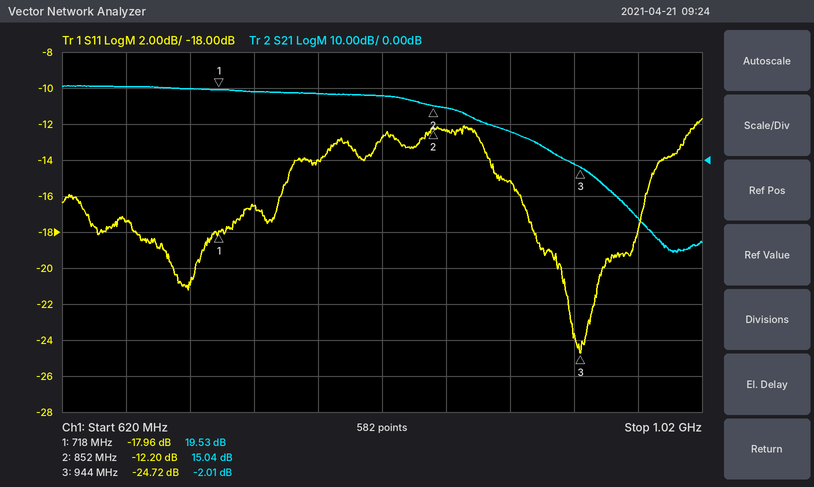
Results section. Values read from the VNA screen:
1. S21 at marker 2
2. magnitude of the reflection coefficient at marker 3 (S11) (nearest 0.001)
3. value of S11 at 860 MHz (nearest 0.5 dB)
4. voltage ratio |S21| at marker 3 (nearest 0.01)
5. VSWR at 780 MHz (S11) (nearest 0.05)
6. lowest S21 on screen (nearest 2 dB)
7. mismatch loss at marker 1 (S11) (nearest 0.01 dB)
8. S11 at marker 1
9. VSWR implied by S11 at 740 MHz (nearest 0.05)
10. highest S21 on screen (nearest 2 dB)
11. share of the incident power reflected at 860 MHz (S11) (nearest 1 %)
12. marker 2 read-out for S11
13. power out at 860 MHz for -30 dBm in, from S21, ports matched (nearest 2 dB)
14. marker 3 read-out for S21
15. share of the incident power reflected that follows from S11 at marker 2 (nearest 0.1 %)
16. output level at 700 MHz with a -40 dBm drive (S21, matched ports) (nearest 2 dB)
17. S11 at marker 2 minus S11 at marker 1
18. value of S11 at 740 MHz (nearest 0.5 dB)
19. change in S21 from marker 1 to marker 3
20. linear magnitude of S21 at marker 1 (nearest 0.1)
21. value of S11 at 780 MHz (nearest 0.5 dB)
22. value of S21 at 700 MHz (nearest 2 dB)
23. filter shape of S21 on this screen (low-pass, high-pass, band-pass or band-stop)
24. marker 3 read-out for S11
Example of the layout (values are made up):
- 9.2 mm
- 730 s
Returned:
- 15.04 dB
- 0.058
- -12.5 dB
- 0.79
- 1.50
- -26 dB
- 0.07 dB
- -17.96 dB
- 1.35
- 20 dB
- 6 %
- -12.20 dB
- -16 dBm
- -2.01 dB
- 6.0 %
- -20 dBm
- 5.76 dB
- -16.5 dB
- -21.54 dB
- 9.5
- -14.0 dB
- 20 dB
- low-pass
- -24.72 dB
